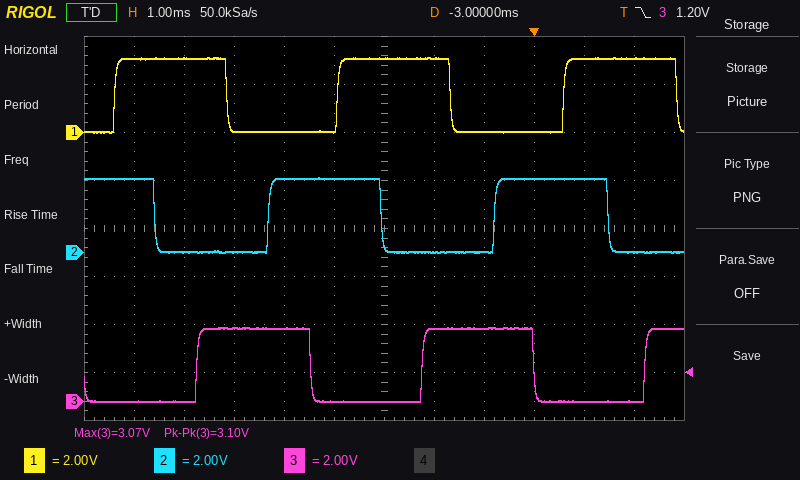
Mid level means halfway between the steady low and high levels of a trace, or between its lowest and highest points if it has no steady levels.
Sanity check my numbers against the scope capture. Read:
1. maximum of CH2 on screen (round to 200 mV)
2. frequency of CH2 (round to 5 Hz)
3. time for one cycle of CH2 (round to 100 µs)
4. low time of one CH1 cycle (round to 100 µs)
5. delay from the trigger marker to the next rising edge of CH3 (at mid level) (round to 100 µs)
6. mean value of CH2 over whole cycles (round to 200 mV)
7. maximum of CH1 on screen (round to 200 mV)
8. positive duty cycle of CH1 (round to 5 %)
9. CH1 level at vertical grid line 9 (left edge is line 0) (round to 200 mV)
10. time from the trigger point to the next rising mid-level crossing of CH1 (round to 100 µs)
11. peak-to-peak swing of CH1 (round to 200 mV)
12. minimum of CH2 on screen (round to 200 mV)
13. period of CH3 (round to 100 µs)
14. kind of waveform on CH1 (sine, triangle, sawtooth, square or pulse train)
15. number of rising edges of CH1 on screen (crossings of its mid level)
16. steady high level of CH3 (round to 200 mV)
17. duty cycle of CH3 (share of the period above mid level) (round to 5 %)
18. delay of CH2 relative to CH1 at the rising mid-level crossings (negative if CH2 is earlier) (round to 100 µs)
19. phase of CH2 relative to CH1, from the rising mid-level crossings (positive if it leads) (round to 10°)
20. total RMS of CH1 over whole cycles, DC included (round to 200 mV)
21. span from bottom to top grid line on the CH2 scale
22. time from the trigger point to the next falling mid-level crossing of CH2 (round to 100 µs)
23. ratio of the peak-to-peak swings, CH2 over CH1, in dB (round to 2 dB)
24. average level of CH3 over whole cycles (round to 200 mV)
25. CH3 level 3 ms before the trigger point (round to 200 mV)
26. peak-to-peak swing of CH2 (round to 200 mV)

3.2 V
220 Hz
4.5 ms
2.2 ms
2.2 ms
1.6 V
3.2 V
50 %
0.0 V
600 µs
3.2 V
0.0 V
4.5 ms
square
3
3.0 V
50 %
-1.4 ms
+110°
2.2 V
16 V
1.5 ms
0 dB
1.6 V
0.0 V
3.2 V
